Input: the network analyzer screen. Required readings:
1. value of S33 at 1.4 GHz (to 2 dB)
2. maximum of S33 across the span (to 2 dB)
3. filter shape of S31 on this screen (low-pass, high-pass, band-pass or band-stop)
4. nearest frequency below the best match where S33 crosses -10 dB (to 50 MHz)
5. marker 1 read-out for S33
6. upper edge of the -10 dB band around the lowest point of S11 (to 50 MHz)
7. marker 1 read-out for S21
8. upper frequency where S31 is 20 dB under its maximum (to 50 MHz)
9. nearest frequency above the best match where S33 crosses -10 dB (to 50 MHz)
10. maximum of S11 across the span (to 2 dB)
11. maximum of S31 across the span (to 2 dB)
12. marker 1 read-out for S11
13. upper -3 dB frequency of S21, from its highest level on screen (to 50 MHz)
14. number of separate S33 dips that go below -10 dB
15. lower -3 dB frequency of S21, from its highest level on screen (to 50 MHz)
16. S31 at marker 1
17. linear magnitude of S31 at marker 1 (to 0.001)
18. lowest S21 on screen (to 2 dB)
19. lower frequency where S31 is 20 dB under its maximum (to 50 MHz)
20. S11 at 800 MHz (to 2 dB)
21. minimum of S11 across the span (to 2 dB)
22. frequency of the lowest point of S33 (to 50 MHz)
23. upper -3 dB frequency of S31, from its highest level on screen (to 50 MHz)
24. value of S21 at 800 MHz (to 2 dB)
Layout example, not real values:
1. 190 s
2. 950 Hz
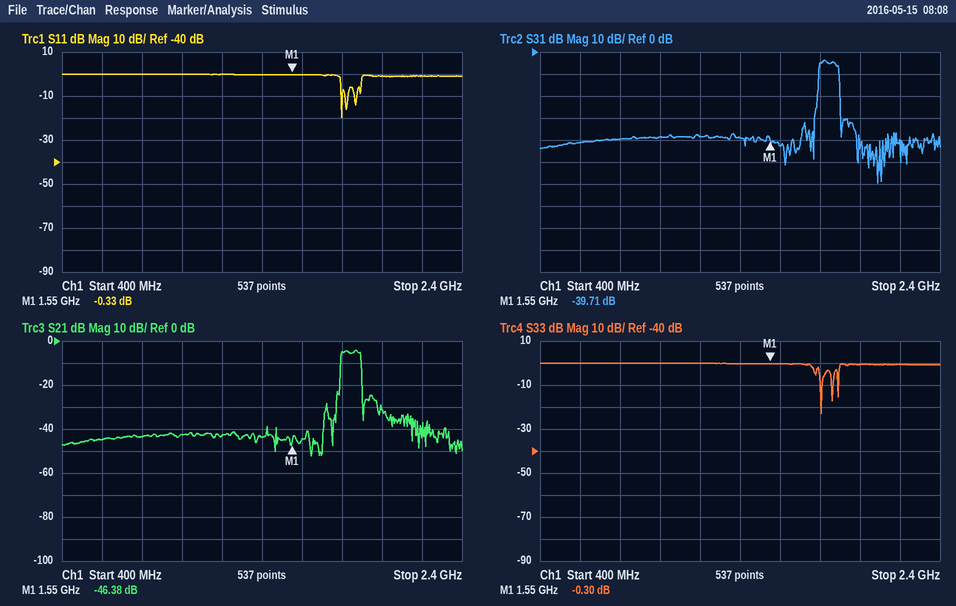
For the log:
1. 0 dB
2. 0 dB
3. band-pass
4. 1.80 GHz
5. -0.30 dB
6. 1.80 GHz
7. -46.38 dB
8. 1.90 GHz
9. 1.80 GHz
10. 0 dB
11. -4 dB
12. -0.33 dB
13. 1.90 GHz
14. 3
15. 1.80 GHz
16. -39.71 dB
17. 0.010
18. -52 dB
19. 1.80 GHz
20. 0 dB
21. -20 dB
22. 1.80 GHz
23. 1.90 GHz
24. -44 dB
